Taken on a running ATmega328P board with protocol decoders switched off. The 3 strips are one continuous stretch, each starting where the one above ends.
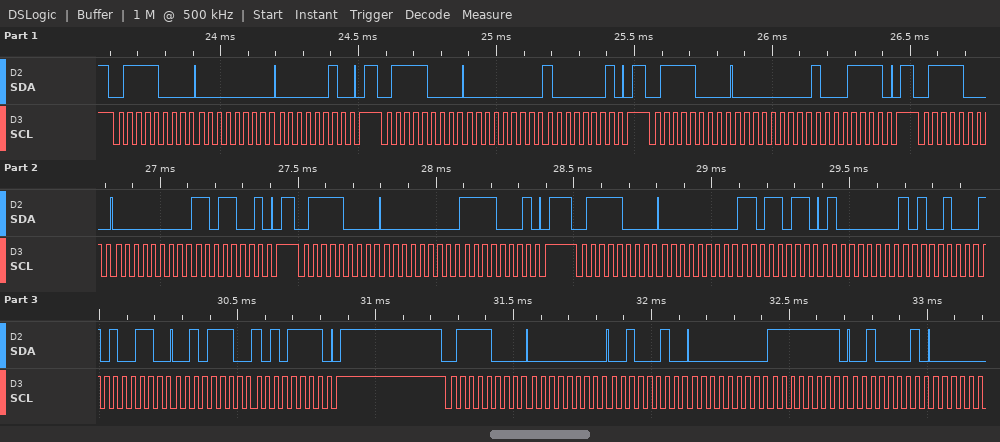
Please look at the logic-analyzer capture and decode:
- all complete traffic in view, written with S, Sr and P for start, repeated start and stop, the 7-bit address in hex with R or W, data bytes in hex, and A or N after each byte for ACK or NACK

S 3CW A 00 A 02 A P S 3CW A 00 A 81 A P S 3CW A 00 A 8F A P S 3CW A 00 A D9 A P S 3CW A 00 A F1 A P S 3CW A 00 A DB A 40 A A4 A A6 A 2E A AF A P S 3CW A 00 A 22 A 00 A FF A 21 A
